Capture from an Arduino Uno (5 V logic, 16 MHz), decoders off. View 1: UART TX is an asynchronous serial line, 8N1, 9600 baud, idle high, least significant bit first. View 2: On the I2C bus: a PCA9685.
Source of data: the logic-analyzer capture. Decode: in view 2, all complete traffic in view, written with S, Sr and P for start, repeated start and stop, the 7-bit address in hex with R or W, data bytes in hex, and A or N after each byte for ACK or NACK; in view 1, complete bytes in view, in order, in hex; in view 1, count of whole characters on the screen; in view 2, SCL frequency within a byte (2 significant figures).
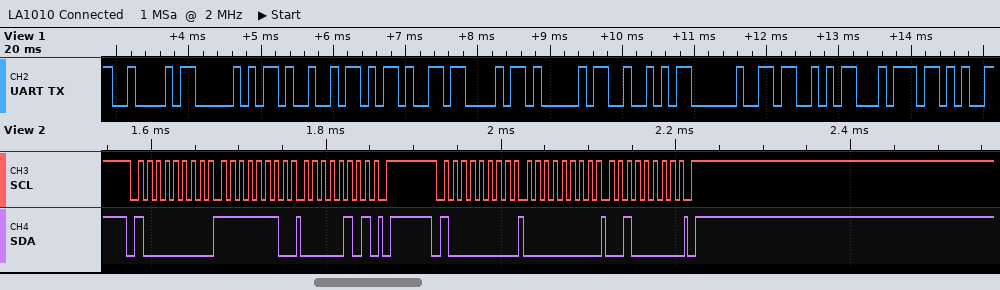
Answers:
S 40W A FE A 05 A P S 40W A 00 A 20 A P
42 50 49 2D 43 41 52 20 53 74
10
100 kHz
